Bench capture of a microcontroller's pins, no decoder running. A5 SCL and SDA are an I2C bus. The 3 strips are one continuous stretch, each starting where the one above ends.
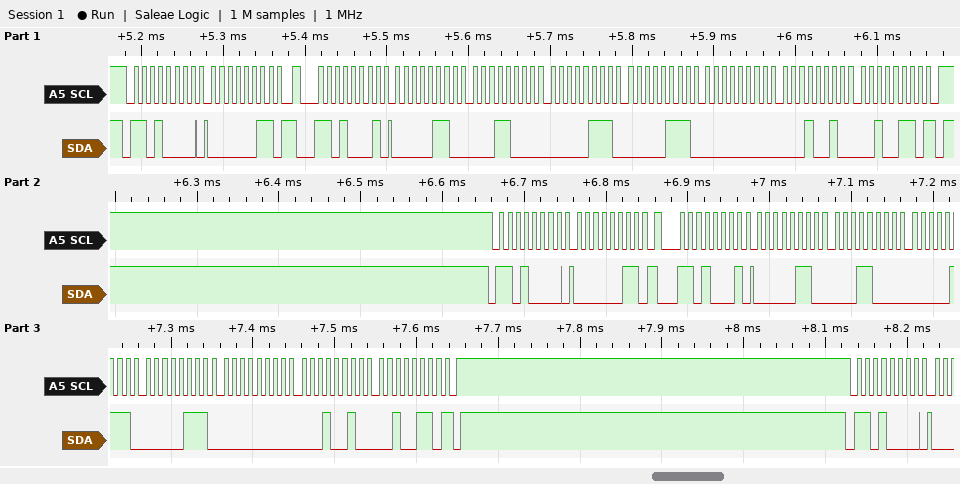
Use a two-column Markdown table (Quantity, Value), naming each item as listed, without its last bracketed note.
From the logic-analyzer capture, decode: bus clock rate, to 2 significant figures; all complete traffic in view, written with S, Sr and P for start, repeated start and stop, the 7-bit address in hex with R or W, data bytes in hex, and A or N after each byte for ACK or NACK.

| Quantity | Value |
|---|---|
| bus clock rate, to 2 significant figures | 100 kHz |
| all complete traffic in view, written with S, Sr and P for start, repeated start and stop, the 7-bit address in hex with R or W, data bytes in hex, and A or N after each byte for ACK or NACK | S 68W A 03 A Sr 68R A 06 A 18 A 07 A 07 A 00 A 12 A 26 N P S 68W A 03 A Sr 68R A 06 A 18 A 07 A 07 A 00 A 12 A 26 N P S 68W A |
